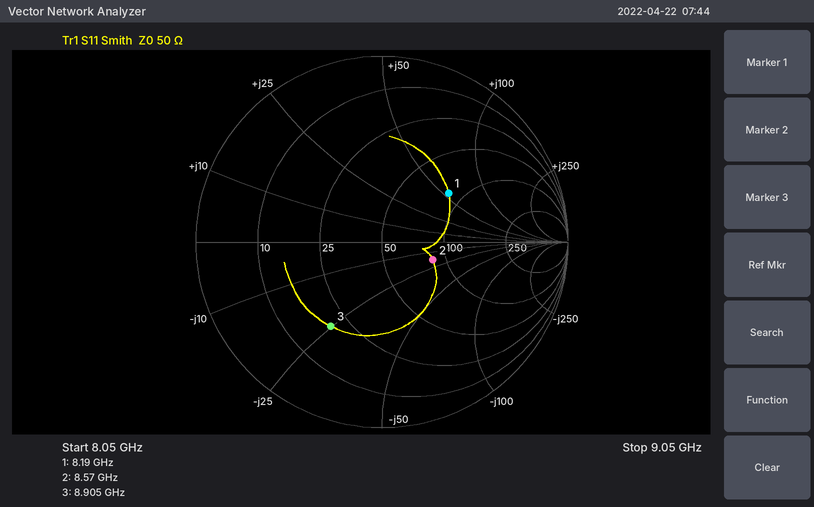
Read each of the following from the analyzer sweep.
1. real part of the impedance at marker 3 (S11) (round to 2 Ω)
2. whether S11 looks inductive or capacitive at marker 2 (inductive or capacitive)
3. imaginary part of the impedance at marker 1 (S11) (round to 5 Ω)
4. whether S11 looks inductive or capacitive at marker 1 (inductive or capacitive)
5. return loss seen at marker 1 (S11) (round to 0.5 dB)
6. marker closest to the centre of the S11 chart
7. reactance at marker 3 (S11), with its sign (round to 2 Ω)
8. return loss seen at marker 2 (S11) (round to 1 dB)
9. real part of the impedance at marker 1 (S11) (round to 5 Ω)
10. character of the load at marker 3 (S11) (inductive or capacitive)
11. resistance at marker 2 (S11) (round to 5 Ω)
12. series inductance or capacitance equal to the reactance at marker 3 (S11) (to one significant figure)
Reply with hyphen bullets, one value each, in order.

- 20 Ω
- capacitive
- +55 Ω
- inductive
- 7.0 dB
- marker 2
- -24 Ω
- 11 dB
- 85 Ω
- capacitive
- 85 Ω
- 700 fF
